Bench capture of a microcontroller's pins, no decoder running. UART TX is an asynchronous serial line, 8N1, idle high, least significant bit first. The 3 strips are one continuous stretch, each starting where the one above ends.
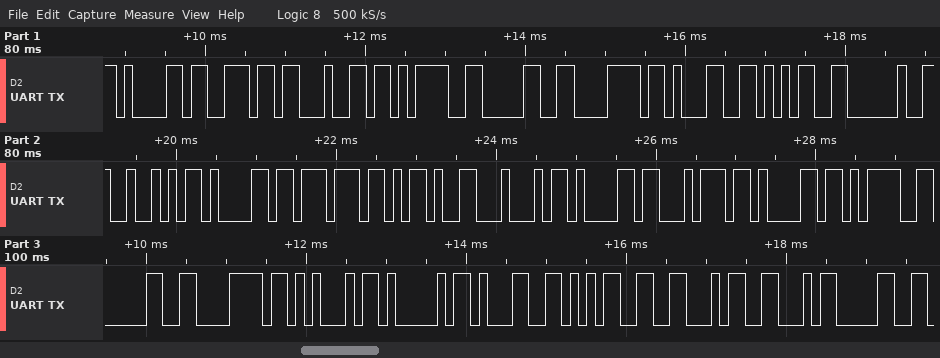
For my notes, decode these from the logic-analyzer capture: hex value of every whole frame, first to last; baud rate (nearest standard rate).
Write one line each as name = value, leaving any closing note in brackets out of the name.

hex value of every whole frame, first to last = 61 6E 64 3D 30 78 31 35 20 52 61 77 2D 44 61 74 61 3D 30 78 45 41 31 35 46 46 30
baud rate = 9600 baud
